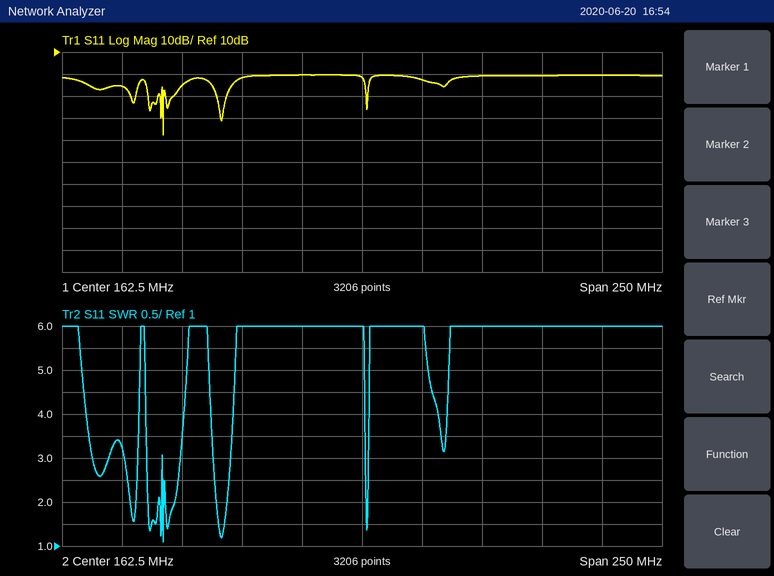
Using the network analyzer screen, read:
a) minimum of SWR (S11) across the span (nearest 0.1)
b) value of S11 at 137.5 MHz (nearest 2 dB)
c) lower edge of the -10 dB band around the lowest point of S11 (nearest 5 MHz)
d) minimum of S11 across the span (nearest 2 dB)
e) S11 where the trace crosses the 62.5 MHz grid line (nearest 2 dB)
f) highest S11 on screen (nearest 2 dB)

1.1
0 dB
80 MHz
-28 dB
-6 dB
0 dB
